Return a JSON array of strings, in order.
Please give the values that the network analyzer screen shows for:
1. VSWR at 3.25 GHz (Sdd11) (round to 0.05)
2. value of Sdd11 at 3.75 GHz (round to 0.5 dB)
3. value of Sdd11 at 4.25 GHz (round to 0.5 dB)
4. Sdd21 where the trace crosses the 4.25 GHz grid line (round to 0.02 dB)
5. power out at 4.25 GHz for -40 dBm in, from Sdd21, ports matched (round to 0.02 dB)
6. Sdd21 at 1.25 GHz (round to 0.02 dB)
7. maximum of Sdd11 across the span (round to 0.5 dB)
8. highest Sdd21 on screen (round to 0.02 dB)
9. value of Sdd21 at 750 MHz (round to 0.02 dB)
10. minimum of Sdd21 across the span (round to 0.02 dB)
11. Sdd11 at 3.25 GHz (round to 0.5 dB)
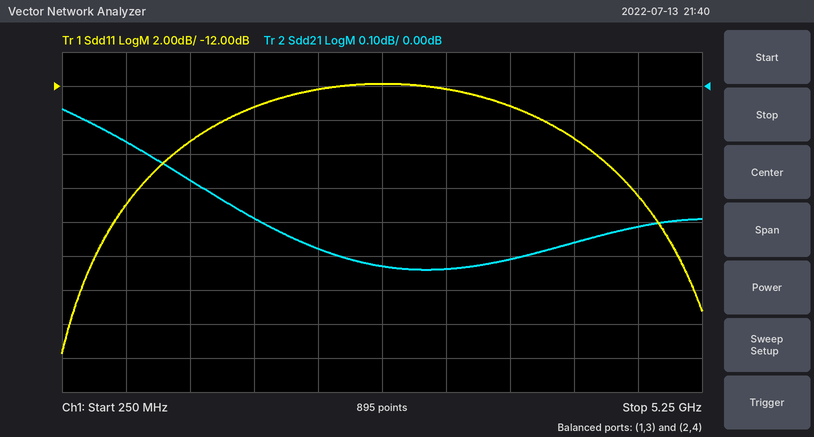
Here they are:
["1.65", "-13.0 dB", "-15.0 dB", "-0.46 dB", "-40.46 dBm", "-0.28 dB", "-12.0 dB", "-0.06 dB", "-0.16 dB", "-0.54 dB", "-12.0 dB"]
